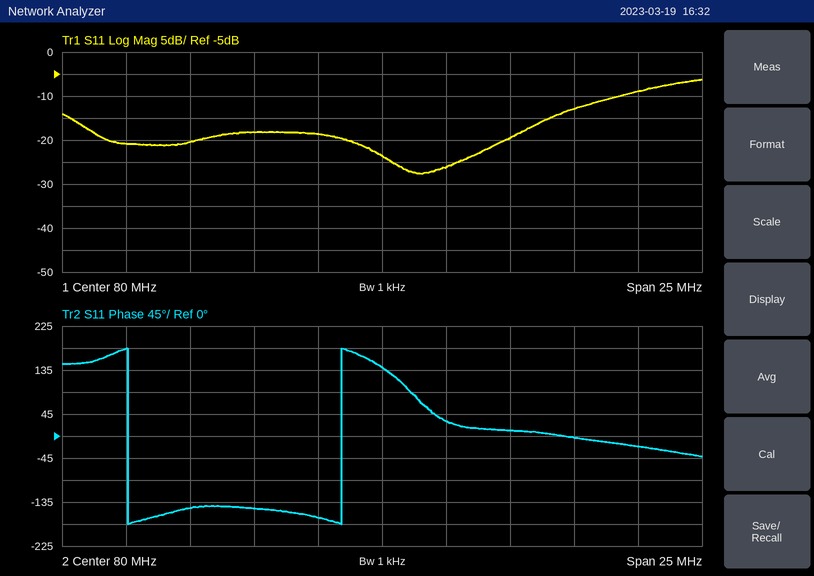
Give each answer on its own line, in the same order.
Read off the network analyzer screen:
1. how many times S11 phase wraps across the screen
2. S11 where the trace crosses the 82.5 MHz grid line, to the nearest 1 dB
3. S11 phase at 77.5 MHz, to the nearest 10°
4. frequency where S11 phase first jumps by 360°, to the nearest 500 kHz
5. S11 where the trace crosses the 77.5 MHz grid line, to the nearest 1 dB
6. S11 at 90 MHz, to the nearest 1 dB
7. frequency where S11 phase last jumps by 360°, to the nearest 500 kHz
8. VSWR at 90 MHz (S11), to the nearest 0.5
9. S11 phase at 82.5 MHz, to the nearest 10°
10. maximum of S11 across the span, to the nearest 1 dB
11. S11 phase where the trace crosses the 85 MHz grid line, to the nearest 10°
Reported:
2
-26 dB
-170°
70.0 MHz
-19 dB
-9 dB
78.5 MHz
2.0
30°
-6 dB
10°
